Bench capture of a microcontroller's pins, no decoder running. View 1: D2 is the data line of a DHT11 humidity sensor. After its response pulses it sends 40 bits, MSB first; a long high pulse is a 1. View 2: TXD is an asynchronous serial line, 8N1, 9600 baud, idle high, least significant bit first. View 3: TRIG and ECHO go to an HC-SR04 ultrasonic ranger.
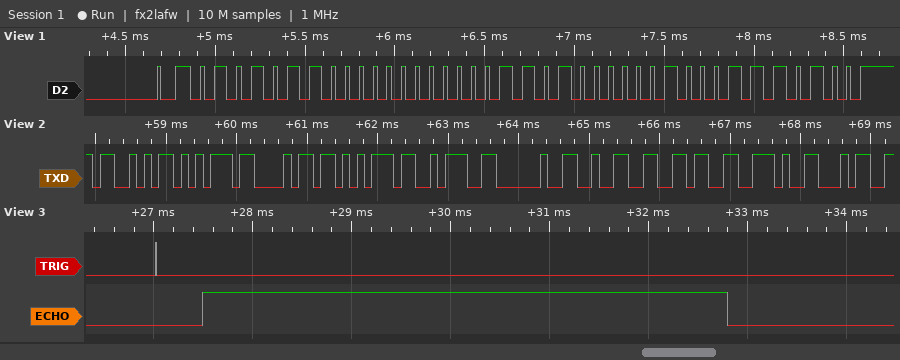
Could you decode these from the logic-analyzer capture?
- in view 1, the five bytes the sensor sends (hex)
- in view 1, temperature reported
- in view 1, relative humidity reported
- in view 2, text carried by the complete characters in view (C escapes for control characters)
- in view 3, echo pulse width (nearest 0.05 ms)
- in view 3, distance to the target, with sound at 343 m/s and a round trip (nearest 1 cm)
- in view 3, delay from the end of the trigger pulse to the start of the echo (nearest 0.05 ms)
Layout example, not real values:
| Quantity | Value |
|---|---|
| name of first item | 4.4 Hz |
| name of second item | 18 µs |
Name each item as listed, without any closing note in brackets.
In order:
| Quantity | Value |
|---|---|
| in view 1, the five bytes the sensor sends | 56 00 1A 04 74 |
| in view 1, temperature reported | 26.4 °C |
| in view 1, relative humidity reported | 86 % |
| in view 2, text carried by the complete characters in view | "Suhu: 26.4" |
| in view 3, echo pulse width | 5.30 ms |
| in view 3, distance to the target, with sound at 343 m/s and a round trip | 91 cm |
| in view 3, delay from the end of the trigger pulse to the start of the echo | 0.45 ms |
